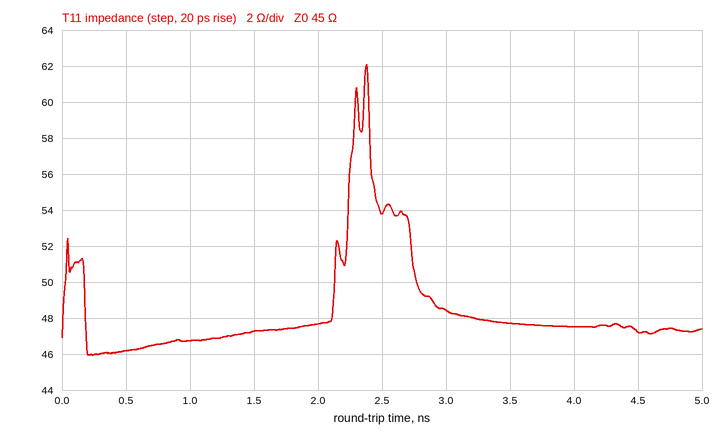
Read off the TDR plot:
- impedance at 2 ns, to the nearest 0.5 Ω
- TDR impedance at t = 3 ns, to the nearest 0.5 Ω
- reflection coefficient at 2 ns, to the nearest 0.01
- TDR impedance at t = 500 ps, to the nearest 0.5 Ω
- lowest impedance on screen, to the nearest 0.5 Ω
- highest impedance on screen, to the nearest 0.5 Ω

47.5 Ω
48.5 Ω
+0.03
46.0 Ω
46.0 Ω
62.0 Ω
